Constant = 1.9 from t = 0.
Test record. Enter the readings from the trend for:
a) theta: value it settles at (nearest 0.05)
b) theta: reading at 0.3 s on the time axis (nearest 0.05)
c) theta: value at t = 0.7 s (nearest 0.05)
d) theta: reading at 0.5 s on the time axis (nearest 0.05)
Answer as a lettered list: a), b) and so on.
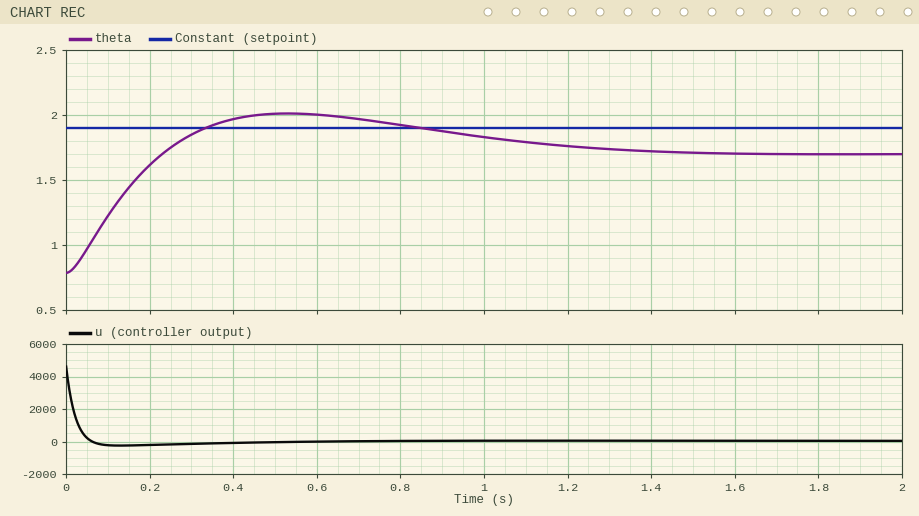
a) 1.70
b) 1.85
c) 1.95
d) 2.00
